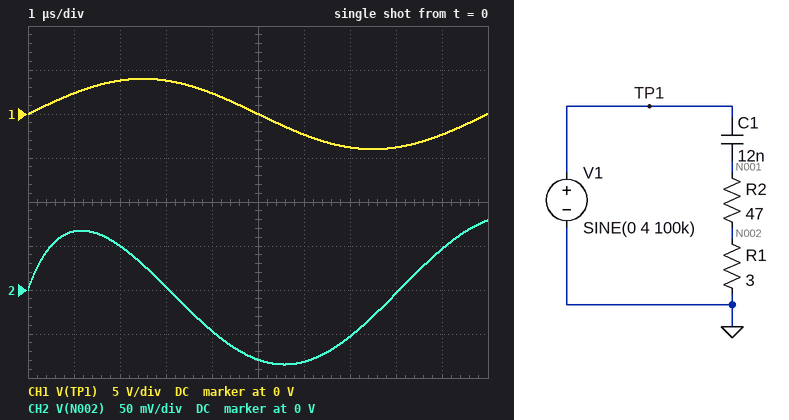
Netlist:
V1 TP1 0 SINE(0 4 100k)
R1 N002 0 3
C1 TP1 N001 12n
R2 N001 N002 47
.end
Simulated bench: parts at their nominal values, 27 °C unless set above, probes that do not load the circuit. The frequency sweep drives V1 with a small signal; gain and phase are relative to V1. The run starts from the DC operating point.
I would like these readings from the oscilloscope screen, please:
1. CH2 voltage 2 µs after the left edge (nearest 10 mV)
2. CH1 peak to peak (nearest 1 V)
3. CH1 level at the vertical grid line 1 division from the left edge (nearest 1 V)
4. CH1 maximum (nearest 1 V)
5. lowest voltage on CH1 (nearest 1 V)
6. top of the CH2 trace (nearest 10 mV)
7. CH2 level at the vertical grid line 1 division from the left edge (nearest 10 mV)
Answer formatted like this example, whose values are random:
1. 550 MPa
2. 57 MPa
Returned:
1. 50 mV
2. 8 V
3. 2 V
4. 4 V
5. -4 V
6. 80 mV
7. 70 mV
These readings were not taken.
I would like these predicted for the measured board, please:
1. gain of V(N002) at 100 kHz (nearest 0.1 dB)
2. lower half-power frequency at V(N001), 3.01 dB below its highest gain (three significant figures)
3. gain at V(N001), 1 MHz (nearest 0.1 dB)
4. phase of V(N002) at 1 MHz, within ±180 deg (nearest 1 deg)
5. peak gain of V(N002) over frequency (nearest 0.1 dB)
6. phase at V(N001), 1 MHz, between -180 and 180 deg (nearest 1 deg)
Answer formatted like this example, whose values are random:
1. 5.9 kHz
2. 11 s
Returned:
1. -33.5 dB
2. 265 kHz
3. -0.3 dB
4. 15 deg
5. -24.4 dB
6. 15 deg
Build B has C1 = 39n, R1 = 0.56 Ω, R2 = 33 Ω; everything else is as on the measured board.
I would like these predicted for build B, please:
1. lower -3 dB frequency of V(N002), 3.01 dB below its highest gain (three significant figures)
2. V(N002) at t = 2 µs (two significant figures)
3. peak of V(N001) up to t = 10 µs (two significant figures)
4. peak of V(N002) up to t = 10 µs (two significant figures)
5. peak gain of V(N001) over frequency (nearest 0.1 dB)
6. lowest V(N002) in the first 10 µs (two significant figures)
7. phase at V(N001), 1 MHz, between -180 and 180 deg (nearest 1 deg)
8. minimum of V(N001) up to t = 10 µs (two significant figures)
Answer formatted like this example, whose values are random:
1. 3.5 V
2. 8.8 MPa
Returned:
1. 122 kHz
2. 29 mV
3. 2.0 V
4. 33 mV
5. 0 dB
6. -43 mV
7. 7 deg
8. -2.6 V
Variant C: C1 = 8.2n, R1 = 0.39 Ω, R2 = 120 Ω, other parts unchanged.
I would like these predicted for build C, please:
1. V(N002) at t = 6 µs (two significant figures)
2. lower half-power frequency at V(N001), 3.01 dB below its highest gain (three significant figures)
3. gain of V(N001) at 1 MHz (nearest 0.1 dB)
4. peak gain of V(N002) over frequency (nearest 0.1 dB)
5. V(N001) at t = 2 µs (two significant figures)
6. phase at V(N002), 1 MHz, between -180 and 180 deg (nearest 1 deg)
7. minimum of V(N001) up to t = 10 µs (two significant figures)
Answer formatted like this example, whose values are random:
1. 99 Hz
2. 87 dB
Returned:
1. -6.8 mV
2. 161 kHz
3. -0.1 dB
4. -49.8 dB
5. 1.4 V
6. 9 deg
7. -2.1 V
